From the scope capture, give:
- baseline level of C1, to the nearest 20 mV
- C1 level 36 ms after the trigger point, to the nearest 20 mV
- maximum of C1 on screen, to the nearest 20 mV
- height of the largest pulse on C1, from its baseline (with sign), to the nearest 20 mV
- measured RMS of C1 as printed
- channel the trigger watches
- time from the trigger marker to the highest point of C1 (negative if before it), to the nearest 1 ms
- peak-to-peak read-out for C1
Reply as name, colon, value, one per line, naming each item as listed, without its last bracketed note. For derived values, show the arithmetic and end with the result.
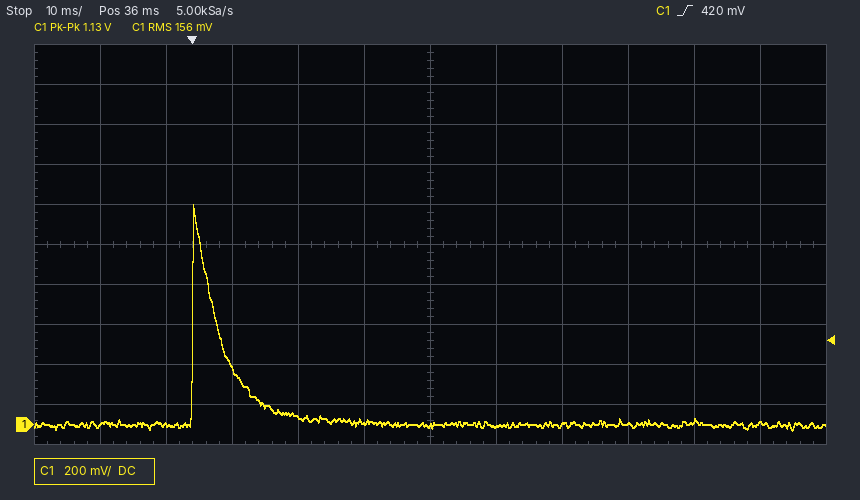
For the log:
baseline level of C1, to the nearest 20 mV: 0 mV
C1 level 36 ms after the trigger point, to the nearest 20 mV: 0 mV
maximum of C1 on screen, to the nearest 20 mV: 1.10 V
height of the largest pulse on C1, from its baseline (with sign), to the nearest 20 mV: 1.10 V − (0 mV) = +1.10 V
measured RMS of C1 as printed: 156 mV
channel the trigger watches: C1
time from the trigger marker to the highest point of C1 (negative if before it), to the nearest 1 ms: 0 ms
peak-to-peak read-out for C1: 1.13 V
